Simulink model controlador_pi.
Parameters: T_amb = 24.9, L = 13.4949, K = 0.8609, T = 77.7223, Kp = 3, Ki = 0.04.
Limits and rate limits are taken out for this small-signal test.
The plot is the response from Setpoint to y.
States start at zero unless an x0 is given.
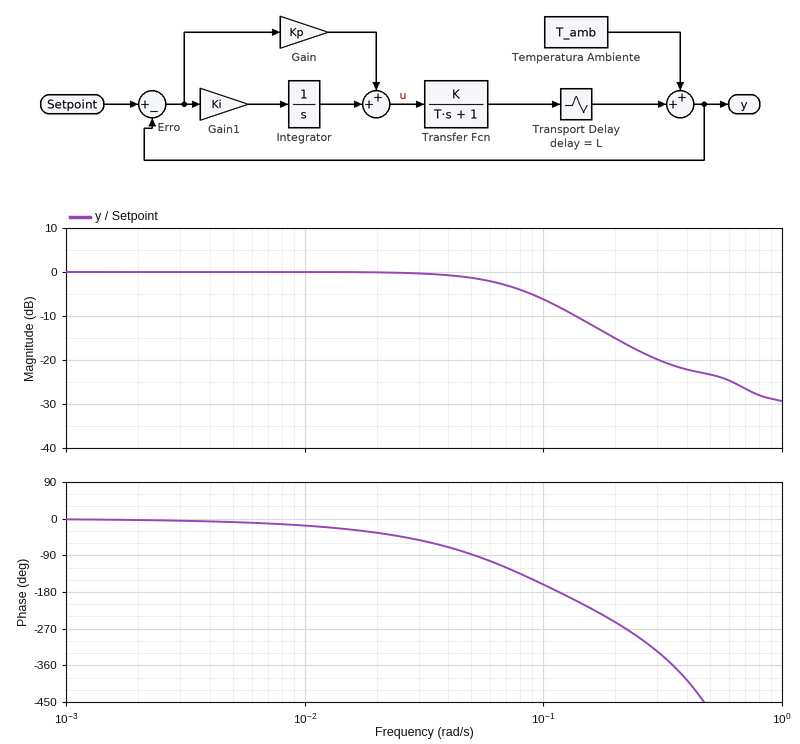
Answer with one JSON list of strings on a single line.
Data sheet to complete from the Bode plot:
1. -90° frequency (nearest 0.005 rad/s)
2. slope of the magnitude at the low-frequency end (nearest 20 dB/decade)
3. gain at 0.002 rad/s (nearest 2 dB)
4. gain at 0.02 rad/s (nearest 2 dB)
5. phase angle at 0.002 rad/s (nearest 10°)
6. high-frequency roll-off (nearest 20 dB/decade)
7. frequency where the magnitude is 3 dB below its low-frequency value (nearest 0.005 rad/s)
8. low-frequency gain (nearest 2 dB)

["0.050 rad/s", "0 dB/decade", "0 dB", "0 dB", "0°", "-20 dB/decade", "0.070 rad/s", "0 dB"]
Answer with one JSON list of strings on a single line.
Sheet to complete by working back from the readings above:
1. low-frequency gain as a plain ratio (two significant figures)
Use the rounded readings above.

["1.0"]
